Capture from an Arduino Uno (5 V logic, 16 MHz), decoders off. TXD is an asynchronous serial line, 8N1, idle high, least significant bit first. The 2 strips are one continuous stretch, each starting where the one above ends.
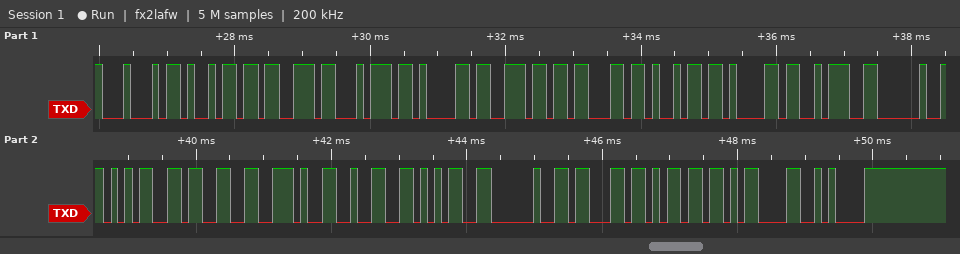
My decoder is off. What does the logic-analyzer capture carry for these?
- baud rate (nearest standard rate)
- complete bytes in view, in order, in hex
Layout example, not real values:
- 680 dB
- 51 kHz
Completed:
- 9600 baud
- 44 69 73 74 61 6E 63 69 61 3A 20 35 33 2E 32 35 20 63 6D 0D 0A
